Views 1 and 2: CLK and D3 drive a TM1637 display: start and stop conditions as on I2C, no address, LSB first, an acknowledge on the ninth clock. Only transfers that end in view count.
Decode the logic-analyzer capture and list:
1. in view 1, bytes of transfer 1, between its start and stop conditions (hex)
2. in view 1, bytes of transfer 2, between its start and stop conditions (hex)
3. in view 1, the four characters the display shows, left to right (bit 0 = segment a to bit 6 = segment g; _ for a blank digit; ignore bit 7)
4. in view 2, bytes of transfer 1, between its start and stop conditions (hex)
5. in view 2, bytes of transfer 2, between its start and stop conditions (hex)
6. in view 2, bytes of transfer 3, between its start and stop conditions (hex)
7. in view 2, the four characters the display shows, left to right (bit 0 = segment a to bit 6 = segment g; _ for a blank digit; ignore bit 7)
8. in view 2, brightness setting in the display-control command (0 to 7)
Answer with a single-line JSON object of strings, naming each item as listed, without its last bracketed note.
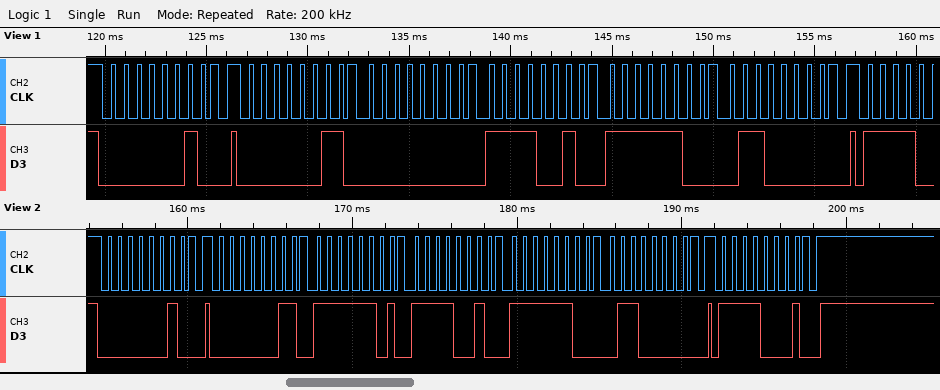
{"in view 1, bytes of transfer 1, between its start and stop conditions": "40", "in view 1, bytes of transfer 2, between its start and stop conditions": "C0 00 4F 3F 06", "in view 1, the four characters the display shows, left to right": "_301", "in view 2, bytes of transfer 1, between its start and stop conditions": "40", "in view 2, bytes of transfer 2, between its start and stop conditions": "C0 BF 4F 3F 06", "in view 2, bytes of transfer 3, between its start and stop conditions": "8F", "in view 2, the four characters the display shows, left to right": "0301", "in view 2, brightness setting in the display-control command": "7"}
